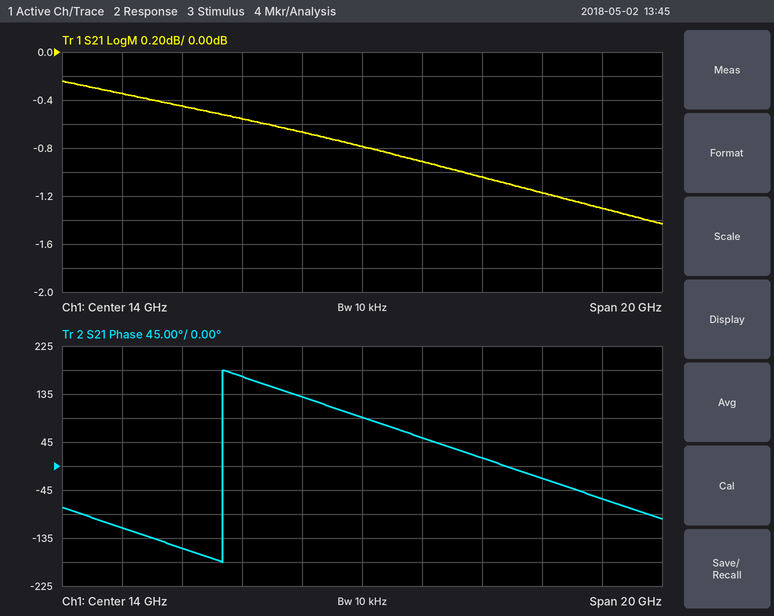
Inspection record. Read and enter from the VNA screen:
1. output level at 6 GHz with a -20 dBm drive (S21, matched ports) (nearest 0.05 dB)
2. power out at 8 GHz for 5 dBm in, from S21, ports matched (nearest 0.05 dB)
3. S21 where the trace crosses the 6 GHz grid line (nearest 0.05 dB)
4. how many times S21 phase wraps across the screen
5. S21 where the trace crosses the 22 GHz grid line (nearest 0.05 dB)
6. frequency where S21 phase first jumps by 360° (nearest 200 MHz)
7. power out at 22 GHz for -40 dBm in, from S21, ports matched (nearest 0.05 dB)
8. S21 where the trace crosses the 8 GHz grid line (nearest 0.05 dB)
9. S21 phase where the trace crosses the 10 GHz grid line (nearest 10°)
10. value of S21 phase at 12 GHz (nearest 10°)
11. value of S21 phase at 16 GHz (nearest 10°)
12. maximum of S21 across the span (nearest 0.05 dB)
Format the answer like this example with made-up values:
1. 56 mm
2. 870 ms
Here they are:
1. -20.35 dBm
2. 4.55 dBm
3. -0.35 dB
4. 1
5. -1.30 dB
6. 9.4 GHz
7. -41.30 dBm
8. -0.45 dB
9. 170°
10. 130°
11. 50°
12. -0.25 dB
